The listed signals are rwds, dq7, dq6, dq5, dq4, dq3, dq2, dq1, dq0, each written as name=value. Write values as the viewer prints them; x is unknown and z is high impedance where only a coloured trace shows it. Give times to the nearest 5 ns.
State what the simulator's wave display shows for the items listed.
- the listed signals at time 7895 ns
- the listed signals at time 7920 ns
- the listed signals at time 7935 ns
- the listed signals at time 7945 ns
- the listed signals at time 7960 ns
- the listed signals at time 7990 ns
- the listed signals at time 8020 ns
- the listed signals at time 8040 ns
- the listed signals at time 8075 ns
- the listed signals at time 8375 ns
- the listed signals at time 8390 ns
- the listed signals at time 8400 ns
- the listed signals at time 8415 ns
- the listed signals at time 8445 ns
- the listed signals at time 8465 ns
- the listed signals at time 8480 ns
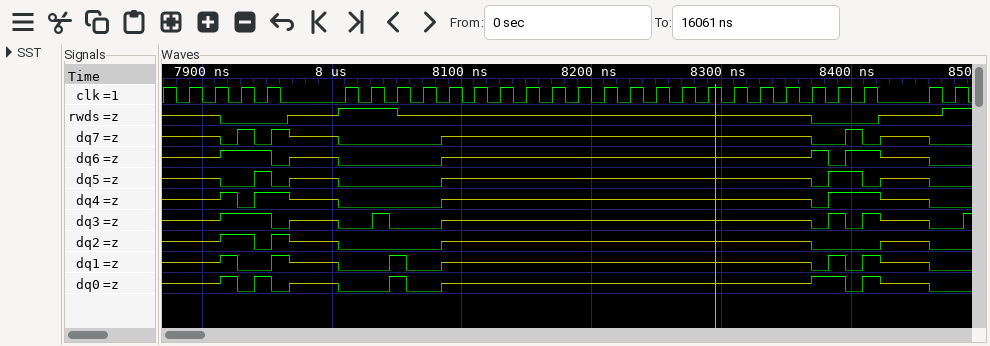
rwds=z, dq7=z, dq6=z, dq5=z, dq4=z, dq3=z, dq2=z, dq1=z, dq0=z
rwds=0, dq7=0, dq6=1, dq5=0, dq4=1, dq3=1, dq2=1, dq1=1, dq0=1
rwds=0, dq7=1, dq6=1, dq5=0, dq4=0, dq3=1, dq2=1, dq1=0, dq0=0
rwds=0, dq7=0, dq6=1, dq5=1, dq4=1, dq3=1, dq2=0, dq1=0, dq0=1
rwds=0, dq7=1, dq6=0, dq5=0, dq4=1, dq3=0, dq2=1, dq1=1, dq0=0
rwds=z, dq7=z, dq6=z, dq5=z, dq4=z, dq3=z, dq2=z, dq1=z, dq0=z
rwds=1, dq7=0, dq6=0, dq5=0, dq4=0, dq3=0, dq2=0, dq1=0, dq0=0
rwds=1, dq7=0, dq6=0, dq5=0, dq4=0, dq3=1, dq2=0, dq1=0, dq0=0
rwds=z, dq7=0, dq6=0, dq5=0, dq4=0, dq3=0, dq2=0, dq1=0, dq0=0
rwds=0, dq7=0, dq6=1, dq5=0, dq4=0, dq3=0, dq2=0, dq1=0, dq0=1
rwds=0, dq7=0, dq6=0, dq5=1, dq4=1, dq3=1, dq2=0, dq1=1, dq0=1
rwds=0, dq7=1, dq6=1, dq5=1, dq4=1, dq3=0, dq2=0, dq1=0, dq0=0
rwds=0, dq7=0, dq6=1, dq5=0, dq4=1, dq3=1, dq2=0, dq1=1, dq0=1
rwds=z, dq7=z, dq6=z, dq5=z, dq4=z, dq3=z, dq2=z, dq1=z, dq0=z
rwds=z, dq7=0, dq6=0, dq5=0, dq4=0, dq3=0, dq2=0, dq1=0, dq0=0
rwds=1, dq7=0, dq6=0, dq5=0, dq4=0, dq3=0, dq2=0, dq1=0, dq0=0
